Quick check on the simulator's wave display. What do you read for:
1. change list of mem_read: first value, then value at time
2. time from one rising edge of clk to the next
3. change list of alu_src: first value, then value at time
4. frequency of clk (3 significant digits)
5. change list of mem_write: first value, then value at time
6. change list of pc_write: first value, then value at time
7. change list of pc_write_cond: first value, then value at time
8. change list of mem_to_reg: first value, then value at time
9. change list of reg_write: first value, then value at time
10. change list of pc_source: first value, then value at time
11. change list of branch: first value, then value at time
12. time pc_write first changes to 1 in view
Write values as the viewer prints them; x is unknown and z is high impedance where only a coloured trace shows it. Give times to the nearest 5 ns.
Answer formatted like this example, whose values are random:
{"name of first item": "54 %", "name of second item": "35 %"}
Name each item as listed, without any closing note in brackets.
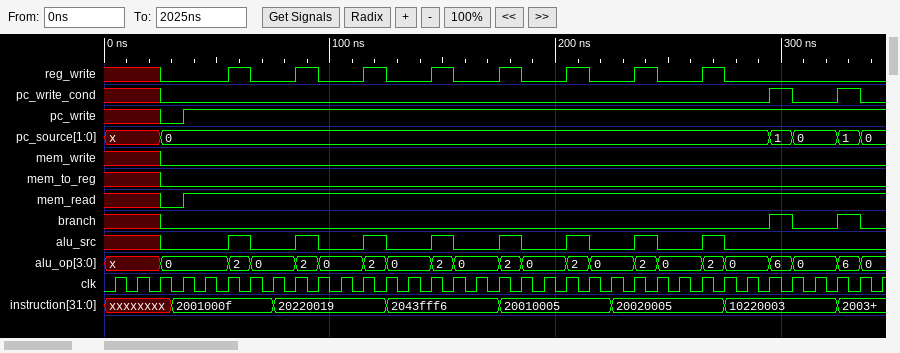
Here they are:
{"change list of mem_read: first value, then value at time": "x, 0 at 25 ns, 1 at 35 ns", "time from one rising edge of clk to the next": "10 ns", "change list of alu_src: first value, then value at time": "x, 0 at 25 ns, 1 at 55 ns, 0 at 65 ns, 1 at 85 ns, 0 at 95 ns, 1 at 115 ns, 0 at 125 ns, 1 at 145 ns, 0 at 155 ns, 1 at 175 ns, 0 at 185 ns, 1 at 205 ns, 0 at 215 ns, 1 at 235 ns, 0 at 245 ns, 1 at 265 ns, 0 at 275 ns", "frequency of clk": "100 MHz", "change list of mem_write: first value, then value at time": "x, 0 at 25 ns", "change list of pc_write: first value, then value at time": "x, 0 at 25 ns, 1 at 35 ns", "change list of pc_write_cond: first value, then value at time": "x, 0 at 25 ns, 1 at 295 ns, 0 at 305 ns, 1 at 325 ns, 0 at 335 ns", "change list of mem_to_reg: first value, then value at time": "x, 0 at 25 ns", "change list of reg_write: first value, then value at time": "x, 0 at 25 ns, 1 at 55 ns, 0 at 65 ns, 1 at 85 ns, 0 at 95 ns, 1 at 115 ns, 0 at 125 ns, 1 at 145 ns, 0 at 155 ns, 1 at 175 ns, 0 at 185 ns, 1 at 205 ns, 0 at 215 ns, 1 at 235 ns, 0 at 245 ns, 1 at 265 ns, 0 at 275 ns", "change list of pc_source: first value, then value at time": "x, 0 at 25 ns, 1 at 295 ns, 0 at 305 ns, 1 at 325 ns, 0 at 335 ns", "change list of branch: first value, then value at time": "x, 0 at 25 ns, 1 at 295 ns, 0 at 305 ns, 1 at 325 ns, 0 at 335 ns", "time pc_write first changes to 1 in view": "35 ns"}
